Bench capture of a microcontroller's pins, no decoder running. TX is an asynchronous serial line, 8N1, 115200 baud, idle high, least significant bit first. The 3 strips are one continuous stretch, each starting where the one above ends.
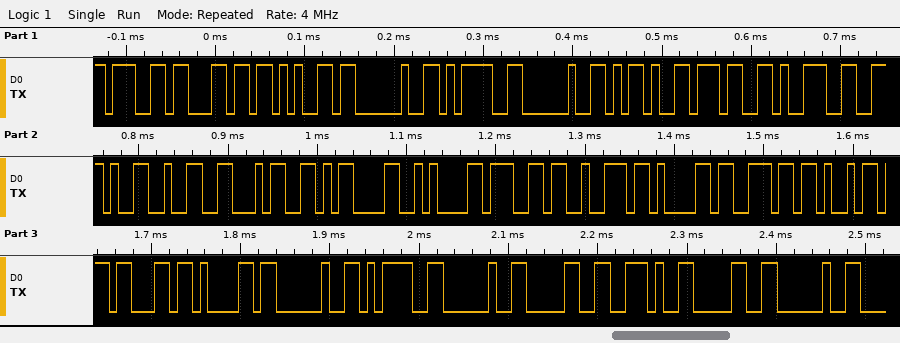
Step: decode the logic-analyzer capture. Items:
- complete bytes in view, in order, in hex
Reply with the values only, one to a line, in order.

67 6C 65 20 3D 20 2D 37 39 2E 32 34 0D 0A 67 72 61 6E 69 63 61 20 3D 20 30 2E 30 20
